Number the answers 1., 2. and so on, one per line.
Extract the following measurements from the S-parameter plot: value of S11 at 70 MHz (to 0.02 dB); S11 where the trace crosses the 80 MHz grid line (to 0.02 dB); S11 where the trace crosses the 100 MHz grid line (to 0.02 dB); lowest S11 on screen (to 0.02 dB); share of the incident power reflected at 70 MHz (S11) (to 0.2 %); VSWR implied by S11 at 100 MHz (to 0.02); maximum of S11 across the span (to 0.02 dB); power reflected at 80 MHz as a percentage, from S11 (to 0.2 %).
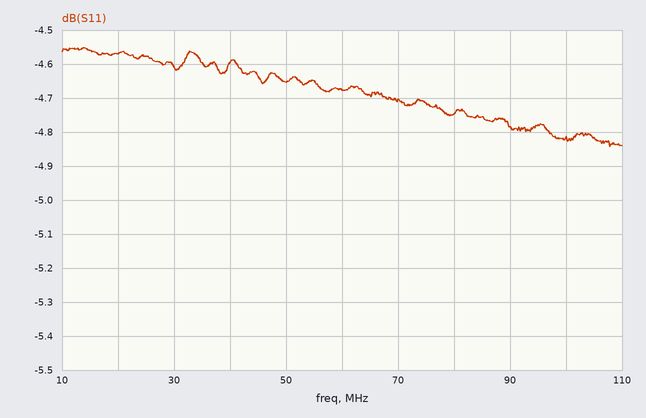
1. -4.70 dB
2. -4.74 dB
3. -4.82 dB
4. -4.84 dB
5. 33.8 %
6. 3.70
7. -4.56 dB
8. 33.6 %
